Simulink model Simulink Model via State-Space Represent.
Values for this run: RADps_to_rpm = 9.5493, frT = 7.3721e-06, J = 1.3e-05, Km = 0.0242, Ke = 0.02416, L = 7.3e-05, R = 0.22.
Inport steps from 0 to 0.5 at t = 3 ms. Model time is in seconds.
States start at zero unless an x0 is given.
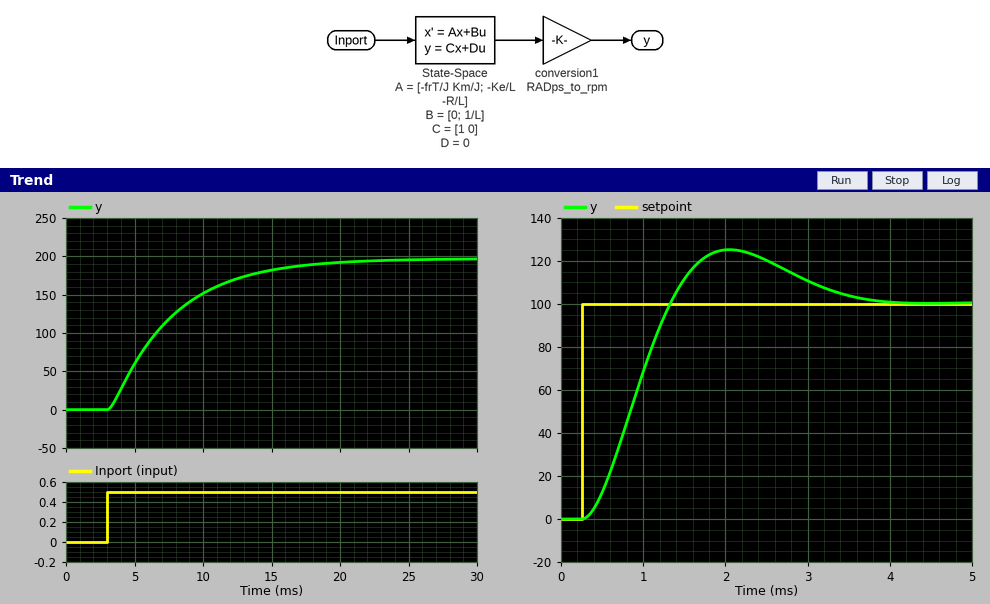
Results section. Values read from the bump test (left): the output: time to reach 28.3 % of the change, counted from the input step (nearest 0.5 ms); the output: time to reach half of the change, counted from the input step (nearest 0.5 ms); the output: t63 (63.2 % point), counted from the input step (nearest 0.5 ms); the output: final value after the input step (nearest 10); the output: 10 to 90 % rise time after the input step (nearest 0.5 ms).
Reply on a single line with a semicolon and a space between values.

2.0 ms; 3.5 ms; 5.0 ms; 200; 10.0 ms
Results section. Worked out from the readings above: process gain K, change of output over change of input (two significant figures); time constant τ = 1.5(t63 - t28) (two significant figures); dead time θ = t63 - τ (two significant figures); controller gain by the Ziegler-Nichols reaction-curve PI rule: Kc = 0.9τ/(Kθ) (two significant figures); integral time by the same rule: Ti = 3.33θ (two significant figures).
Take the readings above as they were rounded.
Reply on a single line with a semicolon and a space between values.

400; 4.5 ms; 0.50 ms; 0.020; 1.7 ms
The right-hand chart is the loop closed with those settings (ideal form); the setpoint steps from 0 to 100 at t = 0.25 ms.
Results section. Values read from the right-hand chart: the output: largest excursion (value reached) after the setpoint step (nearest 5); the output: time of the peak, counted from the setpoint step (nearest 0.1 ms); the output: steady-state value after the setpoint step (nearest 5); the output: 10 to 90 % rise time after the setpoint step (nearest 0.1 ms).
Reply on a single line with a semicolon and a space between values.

125; 1.8 ms; 100; 0.7 ms
